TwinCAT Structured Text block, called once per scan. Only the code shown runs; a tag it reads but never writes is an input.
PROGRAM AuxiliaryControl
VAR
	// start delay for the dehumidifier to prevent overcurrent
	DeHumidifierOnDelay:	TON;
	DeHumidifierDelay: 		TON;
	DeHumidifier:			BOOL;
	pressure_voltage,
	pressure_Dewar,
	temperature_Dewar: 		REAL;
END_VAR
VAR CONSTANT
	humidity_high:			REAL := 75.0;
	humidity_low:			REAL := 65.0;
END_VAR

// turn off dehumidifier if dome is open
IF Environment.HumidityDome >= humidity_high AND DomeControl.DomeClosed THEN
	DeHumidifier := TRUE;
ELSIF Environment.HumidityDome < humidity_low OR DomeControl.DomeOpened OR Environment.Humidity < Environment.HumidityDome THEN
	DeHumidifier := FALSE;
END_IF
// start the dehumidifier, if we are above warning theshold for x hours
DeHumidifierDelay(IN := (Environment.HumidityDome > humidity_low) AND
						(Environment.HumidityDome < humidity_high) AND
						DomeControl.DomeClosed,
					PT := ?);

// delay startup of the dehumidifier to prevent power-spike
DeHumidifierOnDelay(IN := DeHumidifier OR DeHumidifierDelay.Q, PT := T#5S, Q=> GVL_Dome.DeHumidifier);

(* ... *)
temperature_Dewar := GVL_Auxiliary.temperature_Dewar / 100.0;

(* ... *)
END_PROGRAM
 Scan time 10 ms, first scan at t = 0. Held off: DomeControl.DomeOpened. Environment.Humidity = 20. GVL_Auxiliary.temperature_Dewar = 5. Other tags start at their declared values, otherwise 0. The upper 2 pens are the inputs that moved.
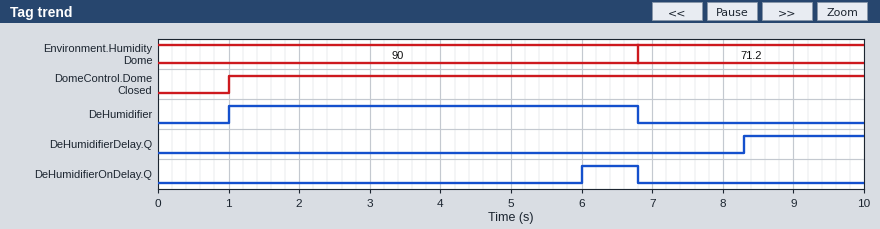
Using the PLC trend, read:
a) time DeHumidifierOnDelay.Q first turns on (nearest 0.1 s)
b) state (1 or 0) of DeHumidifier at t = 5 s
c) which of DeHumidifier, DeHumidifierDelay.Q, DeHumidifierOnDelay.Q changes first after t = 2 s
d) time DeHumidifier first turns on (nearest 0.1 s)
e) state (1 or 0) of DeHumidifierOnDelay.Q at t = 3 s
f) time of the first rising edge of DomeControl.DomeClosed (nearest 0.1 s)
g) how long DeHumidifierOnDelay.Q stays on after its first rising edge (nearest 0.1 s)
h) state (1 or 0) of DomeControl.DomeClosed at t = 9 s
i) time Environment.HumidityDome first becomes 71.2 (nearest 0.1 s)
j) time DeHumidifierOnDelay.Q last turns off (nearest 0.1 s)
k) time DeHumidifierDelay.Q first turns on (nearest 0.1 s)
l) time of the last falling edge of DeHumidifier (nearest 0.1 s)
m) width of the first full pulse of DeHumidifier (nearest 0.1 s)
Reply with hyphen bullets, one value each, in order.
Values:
- 6.0 s
- 1
- DeHumidifierOnDelay.Q
- 1.0 s
- 0
- 1.0 s
- 0.8 s
- 1
- 6.8 s
- 6.8 s
- 8.3 s
- 6.8 s
- 5.8 s
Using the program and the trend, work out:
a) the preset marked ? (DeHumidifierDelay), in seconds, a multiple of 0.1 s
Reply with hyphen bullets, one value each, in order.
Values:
- 1.5 s
